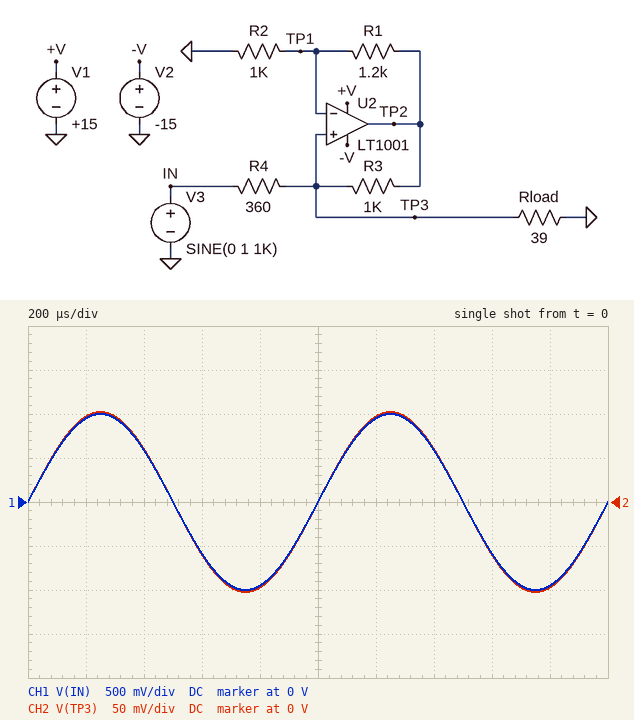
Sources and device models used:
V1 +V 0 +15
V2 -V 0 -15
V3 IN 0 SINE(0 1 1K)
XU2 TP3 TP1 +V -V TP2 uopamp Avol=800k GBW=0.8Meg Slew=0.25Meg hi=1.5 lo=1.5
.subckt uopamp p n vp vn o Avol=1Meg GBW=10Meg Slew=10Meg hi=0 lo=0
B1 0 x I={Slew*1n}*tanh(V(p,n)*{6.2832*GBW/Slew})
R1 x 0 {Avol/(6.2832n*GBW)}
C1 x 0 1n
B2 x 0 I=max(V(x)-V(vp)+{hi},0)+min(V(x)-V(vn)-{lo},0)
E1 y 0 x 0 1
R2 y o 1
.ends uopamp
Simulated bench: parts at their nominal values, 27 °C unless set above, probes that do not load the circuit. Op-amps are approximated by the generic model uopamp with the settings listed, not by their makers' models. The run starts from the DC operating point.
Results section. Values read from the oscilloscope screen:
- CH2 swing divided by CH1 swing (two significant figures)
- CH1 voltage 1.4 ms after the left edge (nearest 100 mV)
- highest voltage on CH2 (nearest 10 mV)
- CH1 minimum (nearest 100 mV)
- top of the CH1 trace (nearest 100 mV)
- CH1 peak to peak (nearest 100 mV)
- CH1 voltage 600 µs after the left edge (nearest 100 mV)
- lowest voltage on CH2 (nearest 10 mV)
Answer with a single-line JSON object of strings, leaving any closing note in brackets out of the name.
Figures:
{"CH2 swing divided by CH1 swing": "0.10", "CH1 voltage 1.4 ms after the left edge": "600 mV", "highest voltage on CH2": "100 mV", "CH1 minimum": "-1.0 V", "top of the CH1 trace": "1.0 V", "CH1 peak to peak": "2.0 V", "CH1 voltage 600 µs after the left edge": "-600 mV", "lowest voltage on CH2": "-100 mV"}
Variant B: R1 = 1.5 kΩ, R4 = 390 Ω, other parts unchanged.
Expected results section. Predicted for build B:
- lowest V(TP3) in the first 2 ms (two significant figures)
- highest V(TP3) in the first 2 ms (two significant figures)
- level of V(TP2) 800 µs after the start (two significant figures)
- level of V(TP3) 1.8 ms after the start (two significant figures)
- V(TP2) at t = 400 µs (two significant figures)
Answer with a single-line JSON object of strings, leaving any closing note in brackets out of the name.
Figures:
{"lowest V(TP3) in the first 2 ms": "-96 mV", "highest V(TP3) in the first 2 ms": "96 mV", "level of V(TP2) 800 µs after the start": "-230 mV", "level of V(TP3) 1.8 ms after the start": "-91 mV", "V(TP2) at t = 400 µs": "140 mV"}
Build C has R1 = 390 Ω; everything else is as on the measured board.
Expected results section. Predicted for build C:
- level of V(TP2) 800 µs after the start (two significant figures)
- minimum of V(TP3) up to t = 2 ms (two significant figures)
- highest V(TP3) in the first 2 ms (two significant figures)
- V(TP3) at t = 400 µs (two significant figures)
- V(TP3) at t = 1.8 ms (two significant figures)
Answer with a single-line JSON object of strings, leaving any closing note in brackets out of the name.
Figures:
{"level of V(TP2) 800 µs after the start": "-130 mV", "minimum of V(TP3) up to t = 2 ms": "-99 mV", "highest V(TP3) in the first 2 ms": "99 mV", "V(TP3) at t = 400 µs": "58 mV", "V(TP3) at t = 1.8 ms": "-94 mV"}
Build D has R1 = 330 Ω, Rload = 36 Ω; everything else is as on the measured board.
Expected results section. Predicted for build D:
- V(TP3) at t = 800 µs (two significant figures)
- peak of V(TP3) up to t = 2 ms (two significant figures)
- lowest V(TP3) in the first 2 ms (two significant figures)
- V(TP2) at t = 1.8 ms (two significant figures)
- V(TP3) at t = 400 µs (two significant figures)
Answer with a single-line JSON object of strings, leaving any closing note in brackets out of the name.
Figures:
{"V(TP3) at t = 800 µs": "-87 mV", "peak of V(TP3) up to t = 2 ms": "92 mV", "lowest V(TP3) in the first 2 ms": "-92 mV", "V(TP2) at t = 1.8 ms": "-120 mV", "V(TP3) at t = 400 µs": "54 mV"}
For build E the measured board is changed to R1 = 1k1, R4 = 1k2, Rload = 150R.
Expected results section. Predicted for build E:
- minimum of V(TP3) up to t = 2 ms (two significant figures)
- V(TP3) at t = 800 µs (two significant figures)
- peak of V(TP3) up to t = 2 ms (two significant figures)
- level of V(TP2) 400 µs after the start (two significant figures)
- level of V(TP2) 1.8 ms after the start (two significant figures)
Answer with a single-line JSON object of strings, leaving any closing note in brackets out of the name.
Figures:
{"minimum of V(TP3) up to t = 2 ms": "-130 mV", "V(TP3) at t = 800 µs": "-120 mV", "peak of V(TP3) up to t = 2 ms": "130 mV", "level of V(TP2) 400 µs after the start": "160 mV", "level of V(TP2) 1.8 ms after the start": "-260 mV"}
